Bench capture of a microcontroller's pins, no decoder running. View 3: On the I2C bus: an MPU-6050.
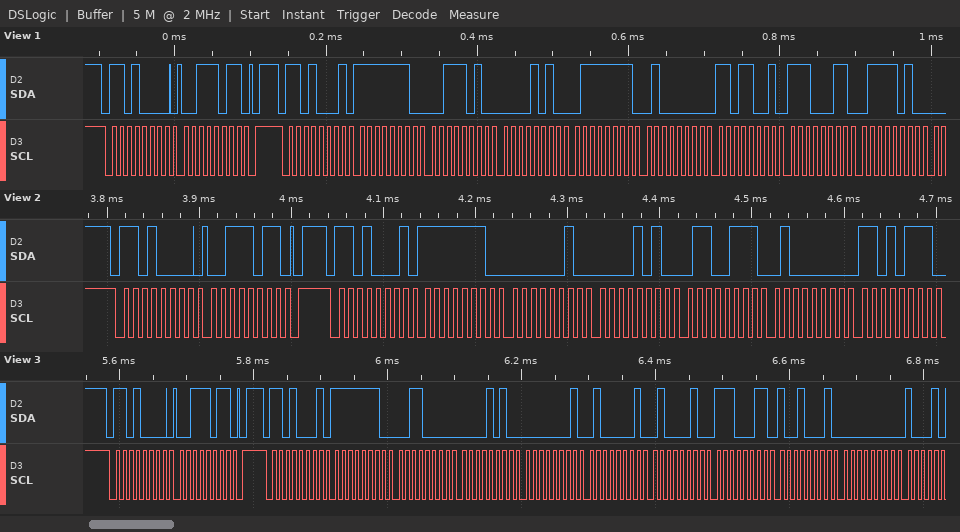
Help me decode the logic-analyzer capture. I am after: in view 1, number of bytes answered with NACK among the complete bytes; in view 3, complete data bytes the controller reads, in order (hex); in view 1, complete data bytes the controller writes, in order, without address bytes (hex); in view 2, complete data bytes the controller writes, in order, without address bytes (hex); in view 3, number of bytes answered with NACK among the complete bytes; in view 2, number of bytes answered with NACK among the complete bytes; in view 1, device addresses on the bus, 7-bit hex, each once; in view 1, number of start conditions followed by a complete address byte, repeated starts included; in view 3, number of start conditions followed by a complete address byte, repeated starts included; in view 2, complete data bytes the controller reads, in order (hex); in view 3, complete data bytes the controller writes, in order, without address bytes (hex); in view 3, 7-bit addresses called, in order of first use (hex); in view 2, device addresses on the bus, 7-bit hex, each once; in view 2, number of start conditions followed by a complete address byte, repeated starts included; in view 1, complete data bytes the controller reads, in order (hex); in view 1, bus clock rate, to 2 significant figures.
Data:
0
FE 30 0A 01 41 42 E3 91 00
3B
3B
0
0
0x68
2
2
FE 02 0A 67 40 D7
3B
0x68
0x68
2
FE 3A 0A 7F 40 D9 E3 7A
100 kHz
